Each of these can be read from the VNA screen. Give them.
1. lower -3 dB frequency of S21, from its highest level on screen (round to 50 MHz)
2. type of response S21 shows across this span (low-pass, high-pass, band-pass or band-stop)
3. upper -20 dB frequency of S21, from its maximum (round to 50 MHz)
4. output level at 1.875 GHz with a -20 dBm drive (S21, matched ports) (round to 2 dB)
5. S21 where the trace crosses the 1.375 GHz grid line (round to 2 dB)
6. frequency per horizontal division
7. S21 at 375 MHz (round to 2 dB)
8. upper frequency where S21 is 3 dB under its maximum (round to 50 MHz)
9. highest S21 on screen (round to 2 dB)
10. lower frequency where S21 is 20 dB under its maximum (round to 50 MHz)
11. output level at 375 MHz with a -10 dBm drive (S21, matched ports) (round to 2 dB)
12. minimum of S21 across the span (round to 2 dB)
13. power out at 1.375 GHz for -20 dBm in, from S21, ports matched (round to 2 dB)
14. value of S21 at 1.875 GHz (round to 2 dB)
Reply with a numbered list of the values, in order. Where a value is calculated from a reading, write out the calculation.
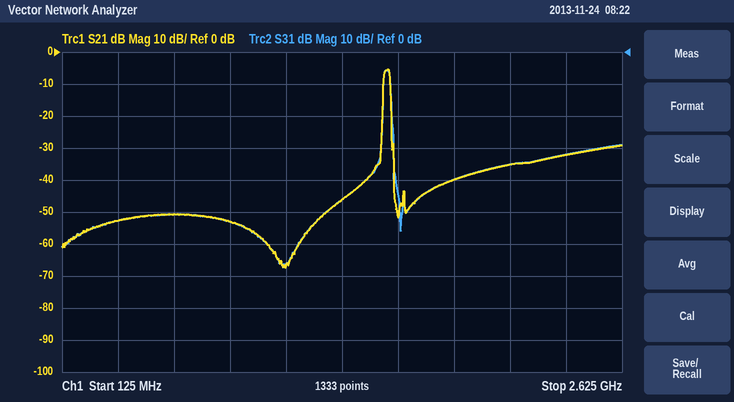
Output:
1. 1.55 GHz
2. band-pass
3. 1.60 GHz
4. -20 dBm + (-40 dB) = -60 dBm
5. -46 dB
6. 250 MHz
7. -52 dB
8. 1.60 GHz
9. -6 dB
10. 1.55 GHz
11. -10 dBm + (-52 dB) = -62 dBm
12. -68 dB
13. -20 dBm + (-46 dB) = -66 dBm
14. -40 dB
